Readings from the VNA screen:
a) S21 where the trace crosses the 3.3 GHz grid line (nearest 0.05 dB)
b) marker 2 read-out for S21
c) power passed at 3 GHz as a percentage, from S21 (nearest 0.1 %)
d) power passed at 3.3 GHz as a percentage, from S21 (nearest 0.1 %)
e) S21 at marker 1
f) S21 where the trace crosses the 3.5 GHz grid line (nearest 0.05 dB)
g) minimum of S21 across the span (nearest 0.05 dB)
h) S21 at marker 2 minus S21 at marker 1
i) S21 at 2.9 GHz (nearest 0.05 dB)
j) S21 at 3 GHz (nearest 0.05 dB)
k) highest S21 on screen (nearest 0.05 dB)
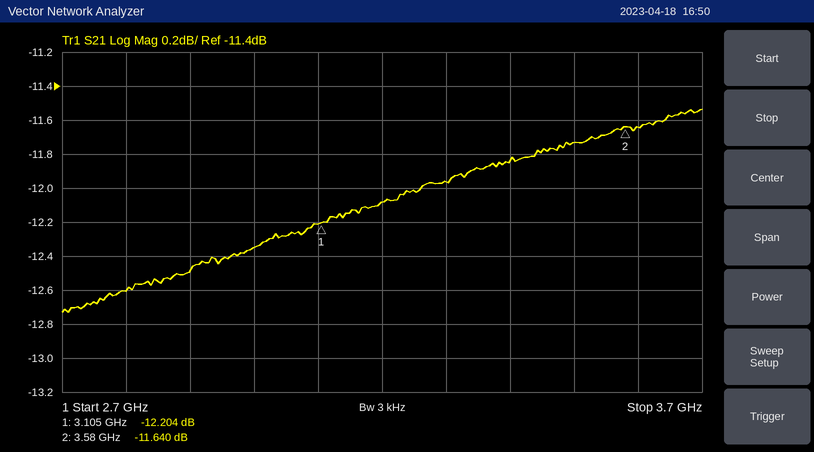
-11.95 dB
-11.640 dB
5.8 %
6.4 %
-12.204 dB
-11.75 dB
-12.75 dB
0.564 dB
-12.50 dB
-12.35 dB
-11.55 dB
